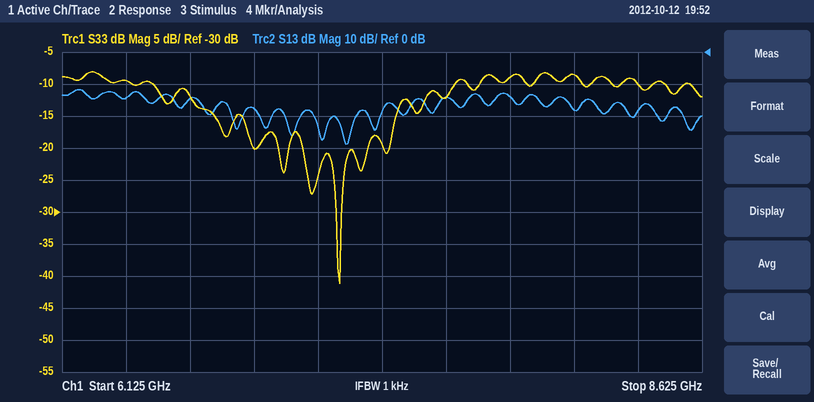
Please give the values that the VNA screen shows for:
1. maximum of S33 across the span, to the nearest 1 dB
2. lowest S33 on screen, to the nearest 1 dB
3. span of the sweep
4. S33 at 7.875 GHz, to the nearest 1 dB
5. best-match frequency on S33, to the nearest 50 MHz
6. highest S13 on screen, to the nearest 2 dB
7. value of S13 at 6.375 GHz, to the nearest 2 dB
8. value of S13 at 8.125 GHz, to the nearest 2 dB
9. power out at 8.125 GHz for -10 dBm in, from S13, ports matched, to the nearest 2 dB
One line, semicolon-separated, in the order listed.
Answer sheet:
-8 dB; -41 dB; 2.5 GHz; -9 dB; 7.20 GHz; -12 dB; -14 dB; -18 dB; -28 dBm
